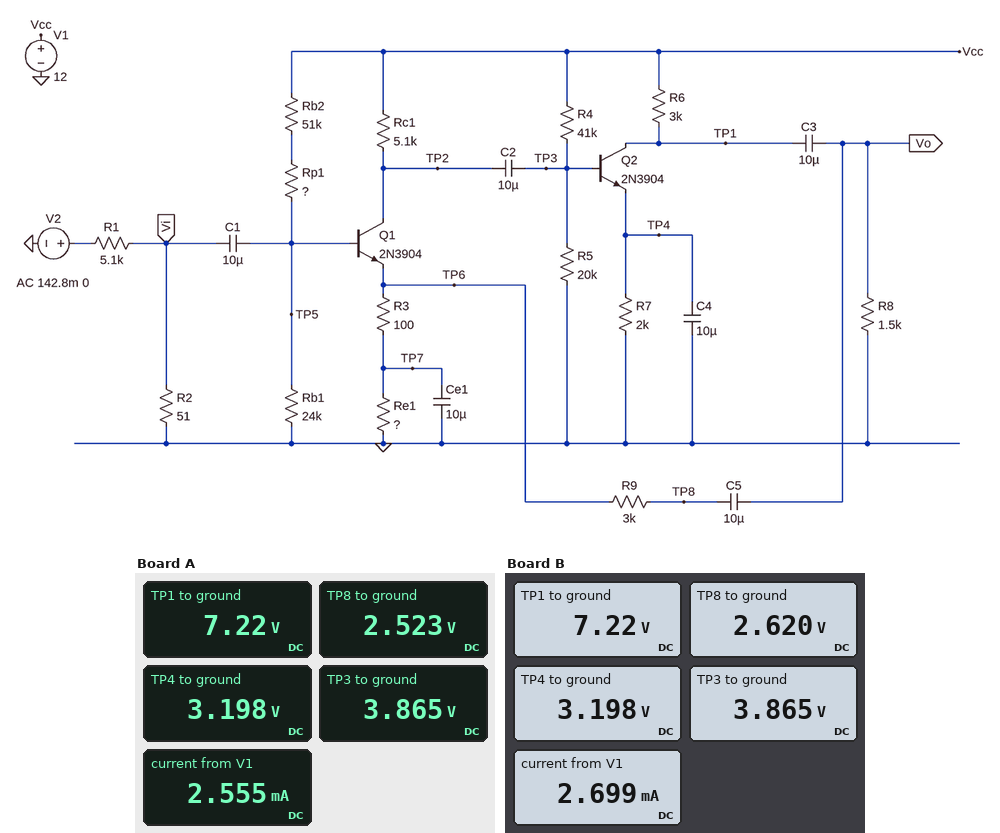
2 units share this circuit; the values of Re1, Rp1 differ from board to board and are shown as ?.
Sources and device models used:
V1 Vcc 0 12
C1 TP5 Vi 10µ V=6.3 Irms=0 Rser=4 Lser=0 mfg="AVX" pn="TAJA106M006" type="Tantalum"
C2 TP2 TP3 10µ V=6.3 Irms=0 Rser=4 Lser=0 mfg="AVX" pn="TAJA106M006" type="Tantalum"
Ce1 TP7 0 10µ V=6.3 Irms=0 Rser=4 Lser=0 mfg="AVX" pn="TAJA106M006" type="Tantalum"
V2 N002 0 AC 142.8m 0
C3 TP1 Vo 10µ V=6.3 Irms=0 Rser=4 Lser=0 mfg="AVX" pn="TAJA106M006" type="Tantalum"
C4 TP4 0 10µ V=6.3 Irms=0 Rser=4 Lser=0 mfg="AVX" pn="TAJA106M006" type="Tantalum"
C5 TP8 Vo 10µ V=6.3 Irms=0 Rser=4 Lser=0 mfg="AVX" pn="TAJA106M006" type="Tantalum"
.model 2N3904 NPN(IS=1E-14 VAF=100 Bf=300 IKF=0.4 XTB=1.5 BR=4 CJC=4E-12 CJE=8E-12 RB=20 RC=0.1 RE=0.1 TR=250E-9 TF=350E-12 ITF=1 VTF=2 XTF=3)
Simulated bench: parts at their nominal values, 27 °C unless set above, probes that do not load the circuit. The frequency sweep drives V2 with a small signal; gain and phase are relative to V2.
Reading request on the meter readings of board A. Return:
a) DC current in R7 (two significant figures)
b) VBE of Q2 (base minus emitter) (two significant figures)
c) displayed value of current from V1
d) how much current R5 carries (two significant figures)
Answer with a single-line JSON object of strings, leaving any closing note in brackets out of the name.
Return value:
{"DC current in R7": "1.6 mA", "VBE of Q2 (base minus emitter)": "670 mV", "displayed value of current from V1": "2.555 mA", "how much current R5 carries": "190 µA"}
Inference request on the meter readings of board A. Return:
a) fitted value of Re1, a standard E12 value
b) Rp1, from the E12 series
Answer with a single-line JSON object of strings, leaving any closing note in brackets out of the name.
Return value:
{"fitted value of Re1, a standard E12 value": "3.9 kΩ", "Rp1, from the E12 series": "15 kΩ"}
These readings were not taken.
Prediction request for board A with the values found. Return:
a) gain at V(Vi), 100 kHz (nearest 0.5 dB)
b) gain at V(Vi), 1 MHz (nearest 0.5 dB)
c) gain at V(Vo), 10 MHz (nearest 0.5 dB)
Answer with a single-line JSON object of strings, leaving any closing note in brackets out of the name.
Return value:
{"gain at V(Vi), 100 kHz": "-40.0 dB", "gain at V(Vi), 1 MHz": "-40.0 dB", "gain at V(Vo), 10 MHz": "-13.0 dB"}
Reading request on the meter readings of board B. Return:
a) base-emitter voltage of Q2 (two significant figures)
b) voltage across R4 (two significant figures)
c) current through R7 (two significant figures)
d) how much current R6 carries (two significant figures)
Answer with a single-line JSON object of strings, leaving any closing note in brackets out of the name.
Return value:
{"base-emitter voltage of Q2": "670 mV", "voltage across R4": "8.1 V", "current through R7": "1.6 mA", "how much current R6 carries": "1.6 mA"}
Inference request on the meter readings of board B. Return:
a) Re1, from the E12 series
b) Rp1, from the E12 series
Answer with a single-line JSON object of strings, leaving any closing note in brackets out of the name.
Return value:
{"Re1, from the E12 series": "3.3 kΩ", "Rp1, from the E12 series": "12 kΩ"}
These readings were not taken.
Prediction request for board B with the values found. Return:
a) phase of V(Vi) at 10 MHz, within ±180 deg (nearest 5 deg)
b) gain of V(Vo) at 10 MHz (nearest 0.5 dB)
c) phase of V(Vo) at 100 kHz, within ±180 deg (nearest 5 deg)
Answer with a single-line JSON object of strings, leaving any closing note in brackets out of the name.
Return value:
{"phase of V(Vi) at 10 MHz, within ±180 deg": "0 deg", "gain of V(Vo) at 10 MHz": "-12.5 dB", "phase of V(Vo) at 100 kHz, within ±180 deg": "0 deg"}
